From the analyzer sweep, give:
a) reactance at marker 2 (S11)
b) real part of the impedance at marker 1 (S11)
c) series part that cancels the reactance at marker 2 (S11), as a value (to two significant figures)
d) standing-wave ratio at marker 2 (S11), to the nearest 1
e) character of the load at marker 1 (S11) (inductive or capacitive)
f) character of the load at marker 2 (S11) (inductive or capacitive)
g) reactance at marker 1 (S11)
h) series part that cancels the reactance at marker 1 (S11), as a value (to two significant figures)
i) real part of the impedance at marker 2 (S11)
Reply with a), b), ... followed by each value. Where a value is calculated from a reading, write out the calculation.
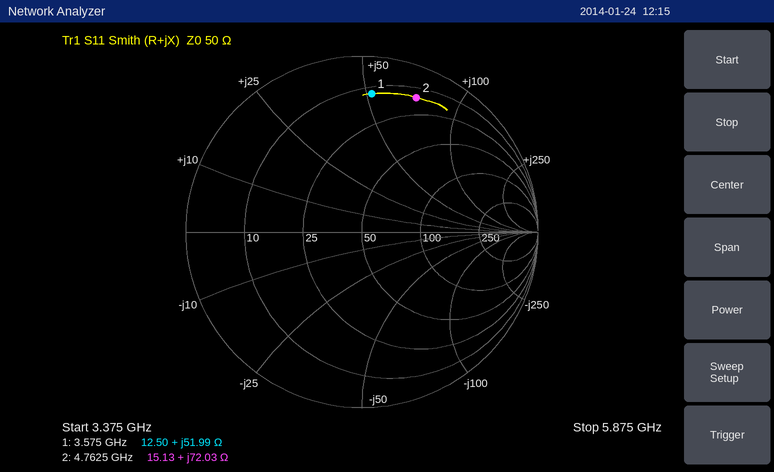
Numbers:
a) +72.03 Ω
b) 12.50 Ω
c) C = 1/(2π × 4.7625 GHz × 72.03 Ω) ≈ 464 fF, so 460 fF to two significant figures
d) 10
e) inductive
f) inductive
g) +51.99 Ω
h) C = 1/(2π × 3.575 GHz × 51.99 Ω) ≈ 856 fF, so 860 fF to two significant figures
i) 15.13 Ω
